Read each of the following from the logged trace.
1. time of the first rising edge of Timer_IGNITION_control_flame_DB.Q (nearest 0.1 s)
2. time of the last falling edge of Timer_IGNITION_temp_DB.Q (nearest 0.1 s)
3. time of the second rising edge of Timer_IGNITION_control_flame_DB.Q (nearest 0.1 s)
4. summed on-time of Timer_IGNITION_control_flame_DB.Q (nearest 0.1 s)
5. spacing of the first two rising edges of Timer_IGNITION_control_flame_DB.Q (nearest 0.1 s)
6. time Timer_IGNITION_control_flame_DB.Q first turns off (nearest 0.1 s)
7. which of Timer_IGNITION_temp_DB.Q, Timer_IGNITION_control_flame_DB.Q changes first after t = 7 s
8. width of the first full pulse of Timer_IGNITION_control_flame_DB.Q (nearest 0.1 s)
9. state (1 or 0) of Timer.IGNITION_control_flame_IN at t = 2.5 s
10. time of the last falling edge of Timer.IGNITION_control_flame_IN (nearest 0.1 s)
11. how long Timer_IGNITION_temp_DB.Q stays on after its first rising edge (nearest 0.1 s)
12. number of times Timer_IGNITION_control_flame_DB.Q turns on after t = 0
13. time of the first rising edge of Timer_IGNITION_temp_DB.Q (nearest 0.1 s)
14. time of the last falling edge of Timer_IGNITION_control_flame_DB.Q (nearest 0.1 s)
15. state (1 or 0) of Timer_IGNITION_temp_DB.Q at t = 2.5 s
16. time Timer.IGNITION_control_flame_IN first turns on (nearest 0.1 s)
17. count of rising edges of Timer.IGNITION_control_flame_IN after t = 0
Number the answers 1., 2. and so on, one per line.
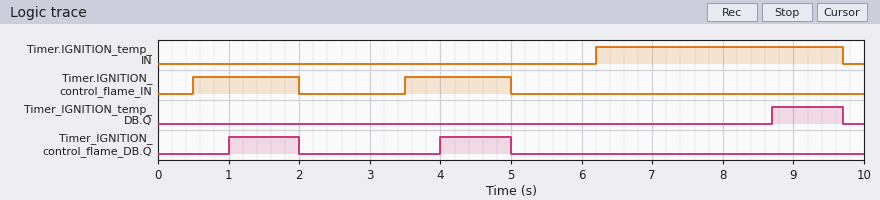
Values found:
1. 1.0 s
2. 9.7 s
3. 4.0 s
4. 2.0 s
5. 3.0 s
6. 2.0 s
7. Timer_IGNITION_temp_DB.Q
8. 1.0 s
9. 0
10. 5.0 s
11. 1.0 s
12. 2
13. 8.7 s
14. 5.0 s
15. 0
16. 0.5 s
17. 2
